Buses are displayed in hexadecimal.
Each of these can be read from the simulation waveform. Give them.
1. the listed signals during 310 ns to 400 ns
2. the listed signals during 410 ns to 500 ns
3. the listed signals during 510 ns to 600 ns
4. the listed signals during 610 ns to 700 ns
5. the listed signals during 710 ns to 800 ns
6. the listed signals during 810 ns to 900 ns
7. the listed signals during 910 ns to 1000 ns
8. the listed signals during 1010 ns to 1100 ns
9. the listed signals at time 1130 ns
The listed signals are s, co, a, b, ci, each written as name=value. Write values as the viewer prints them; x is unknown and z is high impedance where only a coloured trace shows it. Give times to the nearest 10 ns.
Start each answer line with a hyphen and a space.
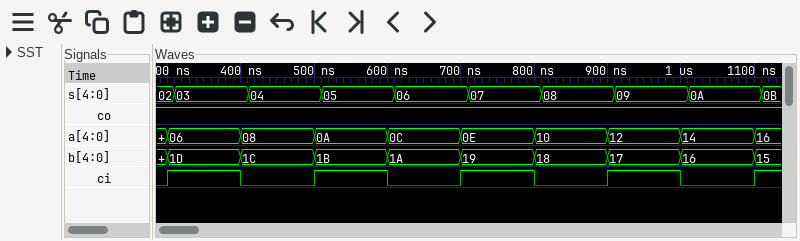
- s=03, co=1, a=06, b=1D, ci=1
- s=04, co=1, a=08, b=1C, ci=0
- s=05, co=1, a=0A, b=1B, ci=1
- s=06, co=1, a=0C, b=1A, ci=0
- s=07, co=1, a=0E, b=19, ci=1
- s=08, co=1, a=10, b=18, ci=0
- s=09, co=1, a=12, b=17, ci=1
- s=0A, co=1, a=14, b=16, ci=0
- s=0B, co=1, a=16, b=15, ci=1
